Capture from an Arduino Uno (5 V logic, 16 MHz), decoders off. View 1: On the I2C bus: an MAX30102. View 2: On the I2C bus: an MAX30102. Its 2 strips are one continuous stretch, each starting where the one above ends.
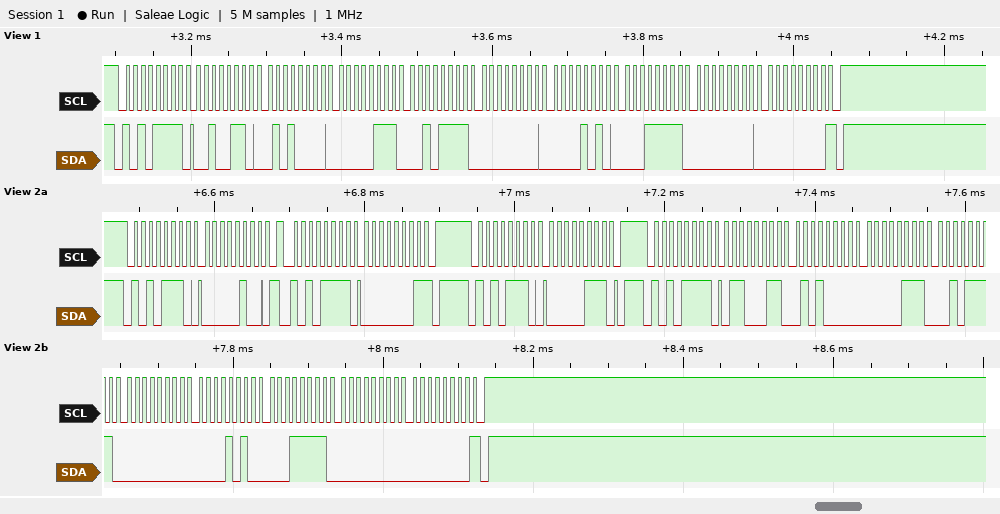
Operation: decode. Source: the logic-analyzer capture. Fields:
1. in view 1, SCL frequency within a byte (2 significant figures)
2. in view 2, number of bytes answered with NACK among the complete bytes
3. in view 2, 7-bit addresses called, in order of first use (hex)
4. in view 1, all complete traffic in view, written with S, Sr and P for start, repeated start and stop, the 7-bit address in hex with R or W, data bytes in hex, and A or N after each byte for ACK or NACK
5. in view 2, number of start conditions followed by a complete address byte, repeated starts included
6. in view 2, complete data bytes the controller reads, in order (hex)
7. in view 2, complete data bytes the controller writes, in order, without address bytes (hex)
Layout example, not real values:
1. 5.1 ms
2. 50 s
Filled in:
1. 100 kHz
2. 2
3. 0x57
4. S 57R A 26 A 50 A 07 A 2F A 00 A 0A A 1F A 00 A 00 N P
5. 4
6. 01 63 50 07 2F 00 0A 1F 00 00
7. 04 07
